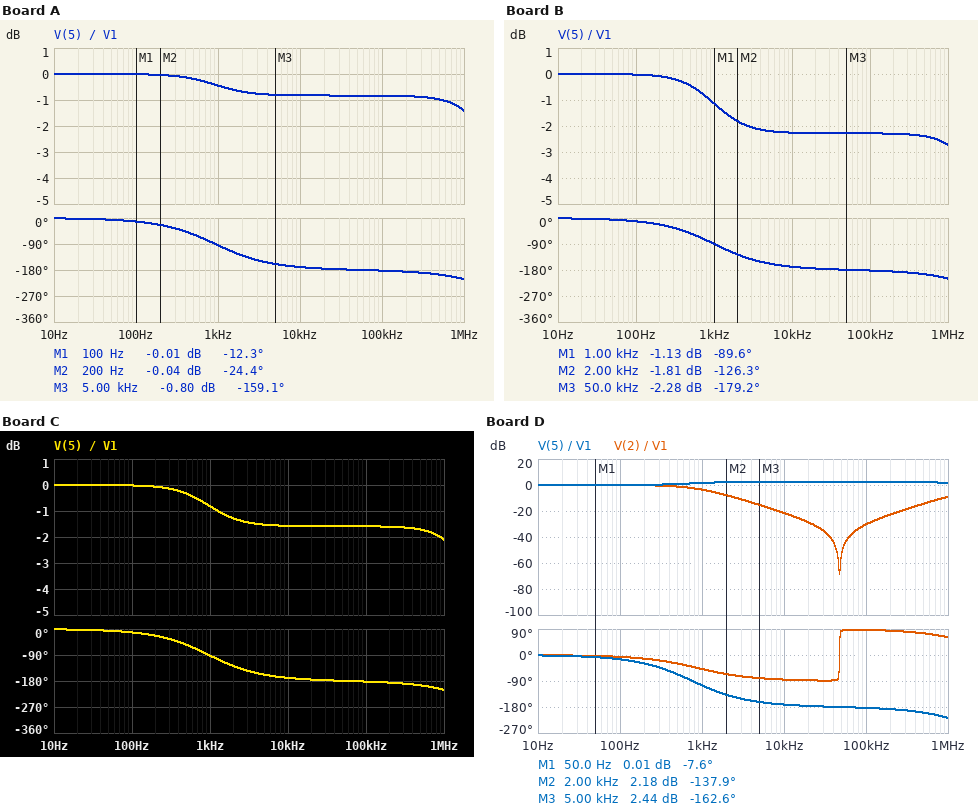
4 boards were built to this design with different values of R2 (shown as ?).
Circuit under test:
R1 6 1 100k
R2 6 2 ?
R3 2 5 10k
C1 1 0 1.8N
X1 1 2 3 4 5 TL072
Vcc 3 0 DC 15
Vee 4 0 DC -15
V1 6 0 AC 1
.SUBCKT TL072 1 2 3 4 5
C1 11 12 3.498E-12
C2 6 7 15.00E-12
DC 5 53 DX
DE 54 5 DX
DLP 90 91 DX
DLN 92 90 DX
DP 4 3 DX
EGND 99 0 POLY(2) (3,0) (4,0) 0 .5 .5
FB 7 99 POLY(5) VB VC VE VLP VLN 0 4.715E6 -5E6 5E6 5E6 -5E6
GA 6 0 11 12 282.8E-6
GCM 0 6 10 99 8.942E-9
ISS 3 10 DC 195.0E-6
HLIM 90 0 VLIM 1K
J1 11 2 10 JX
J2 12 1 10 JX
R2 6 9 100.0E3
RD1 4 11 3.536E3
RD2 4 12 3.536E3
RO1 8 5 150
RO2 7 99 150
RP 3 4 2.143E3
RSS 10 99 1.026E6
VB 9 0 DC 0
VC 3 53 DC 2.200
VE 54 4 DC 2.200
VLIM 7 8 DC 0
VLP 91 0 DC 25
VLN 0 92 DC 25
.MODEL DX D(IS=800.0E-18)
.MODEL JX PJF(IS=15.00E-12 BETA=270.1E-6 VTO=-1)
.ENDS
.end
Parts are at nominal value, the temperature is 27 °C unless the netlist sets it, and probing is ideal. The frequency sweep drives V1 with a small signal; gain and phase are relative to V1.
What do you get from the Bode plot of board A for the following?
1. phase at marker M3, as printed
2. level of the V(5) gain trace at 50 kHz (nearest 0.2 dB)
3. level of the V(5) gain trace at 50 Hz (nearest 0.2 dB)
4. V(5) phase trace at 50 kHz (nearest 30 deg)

-159.1 deg
-0.8 dB
0 dB
-180 deg
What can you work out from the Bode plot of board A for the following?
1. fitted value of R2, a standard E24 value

11 kΩ
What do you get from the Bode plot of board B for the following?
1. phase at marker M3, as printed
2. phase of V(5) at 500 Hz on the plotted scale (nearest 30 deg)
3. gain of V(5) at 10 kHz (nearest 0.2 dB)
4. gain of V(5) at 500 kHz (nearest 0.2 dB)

-179.2 deg
-60 deg
-2.2 dB
-2.4 dB
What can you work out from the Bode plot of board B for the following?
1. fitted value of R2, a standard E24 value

13 kΩ
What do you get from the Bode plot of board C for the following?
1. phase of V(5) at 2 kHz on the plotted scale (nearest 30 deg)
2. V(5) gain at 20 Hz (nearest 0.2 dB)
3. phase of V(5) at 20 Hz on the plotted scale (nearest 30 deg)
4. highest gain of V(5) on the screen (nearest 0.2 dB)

-120 deg
0 dB
0 deg
0 dB
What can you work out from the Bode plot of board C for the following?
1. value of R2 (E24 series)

12 kΩ
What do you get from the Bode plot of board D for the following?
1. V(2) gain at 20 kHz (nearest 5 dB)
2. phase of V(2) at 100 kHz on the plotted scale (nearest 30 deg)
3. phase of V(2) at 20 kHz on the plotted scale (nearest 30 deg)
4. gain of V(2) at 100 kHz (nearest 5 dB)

-30 dB
90 deg
-90 deg
-30 dB
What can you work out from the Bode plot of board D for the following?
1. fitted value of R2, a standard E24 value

7.5 kΩ
